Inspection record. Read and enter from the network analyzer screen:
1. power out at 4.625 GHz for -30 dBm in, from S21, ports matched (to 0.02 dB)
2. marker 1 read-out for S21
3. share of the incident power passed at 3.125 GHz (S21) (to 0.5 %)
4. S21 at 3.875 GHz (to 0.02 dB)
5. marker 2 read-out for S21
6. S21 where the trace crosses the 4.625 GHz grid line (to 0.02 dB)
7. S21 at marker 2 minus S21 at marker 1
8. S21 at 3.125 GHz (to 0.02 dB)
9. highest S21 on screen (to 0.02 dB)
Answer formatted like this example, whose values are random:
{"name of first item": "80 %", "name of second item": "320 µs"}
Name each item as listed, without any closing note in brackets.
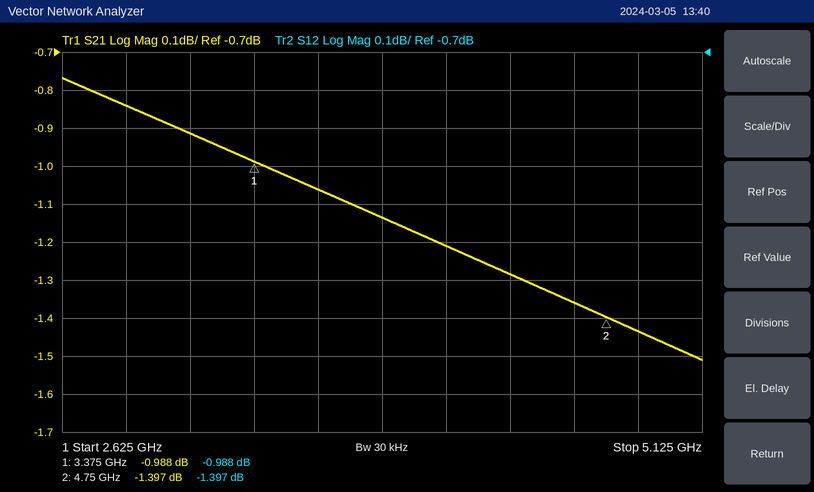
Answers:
{"power out at 4.625 GHz for -30 dBm in, from S21, ports matched": "-31.36 dBm", "marker 1 read-out for S21": "-0.988 dB", "share of the incident power passed at 3.125 GHz (S21)": "81.0 %", "S21 at 3.875 GHz": "-1.14 dB", "marker 2 read-out for S21": "-1.397 dB", "S21 where the trace crosses the 4.625 GHz grid line": "-1.36 dB", "S21 at marker 2 minus S21 at marker 1": "-0.409 dB", "S21 at 3.125 GHz": "-0.92 dB", "highest S21 on screen": "-0.76 dB"}
